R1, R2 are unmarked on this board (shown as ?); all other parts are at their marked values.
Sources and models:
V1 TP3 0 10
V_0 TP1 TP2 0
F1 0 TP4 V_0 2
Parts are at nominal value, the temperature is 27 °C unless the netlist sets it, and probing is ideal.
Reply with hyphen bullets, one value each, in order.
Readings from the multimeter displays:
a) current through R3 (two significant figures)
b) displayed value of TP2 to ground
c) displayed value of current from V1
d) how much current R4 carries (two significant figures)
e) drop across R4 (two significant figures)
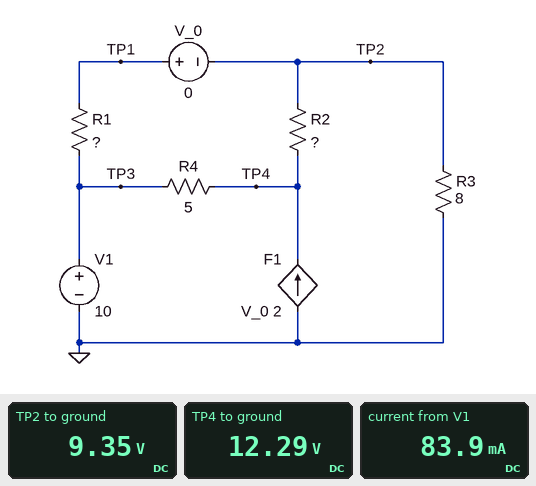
- 1.2 A
- 9.35 V
- 83.9 mA
- 460 mA
- 2.3 V
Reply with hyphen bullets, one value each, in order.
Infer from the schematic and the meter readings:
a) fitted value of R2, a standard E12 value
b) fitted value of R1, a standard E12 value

- 4.7 Ω
- 1.2 Ω
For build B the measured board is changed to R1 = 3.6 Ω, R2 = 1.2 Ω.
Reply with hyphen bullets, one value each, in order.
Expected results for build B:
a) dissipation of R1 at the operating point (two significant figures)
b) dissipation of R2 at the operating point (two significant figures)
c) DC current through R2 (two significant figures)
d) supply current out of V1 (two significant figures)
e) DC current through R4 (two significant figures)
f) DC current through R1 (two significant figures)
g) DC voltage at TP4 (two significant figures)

- 420 mW
- 680 mW
- 750 mA
- 410 mA
- 66 mA
- 340 mA
- 9.7 V
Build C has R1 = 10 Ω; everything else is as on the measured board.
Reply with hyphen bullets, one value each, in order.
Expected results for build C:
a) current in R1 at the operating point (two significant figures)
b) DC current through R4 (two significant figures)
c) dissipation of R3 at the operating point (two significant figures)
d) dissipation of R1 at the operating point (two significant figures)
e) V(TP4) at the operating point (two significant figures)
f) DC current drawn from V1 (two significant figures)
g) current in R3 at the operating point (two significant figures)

- 290 mA
- 18 mA
- 6.3 W
- 840 mW
- 9.9 V
- 310 mA
- 890 mA
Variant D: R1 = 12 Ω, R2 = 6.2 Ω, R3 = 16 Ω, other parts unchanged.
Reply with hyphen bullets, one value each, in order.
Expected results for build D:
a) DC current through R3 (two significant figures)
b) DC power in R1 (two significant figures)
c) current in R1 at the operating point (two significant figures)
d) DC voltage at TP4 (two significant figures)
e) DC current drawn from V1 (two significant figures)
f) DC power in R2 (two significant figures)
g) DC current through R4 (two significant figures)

- 500 mA
- 340 mW
- 170 mA
- 10 V
- 160 mA
- 680 mW
- 6.0 mA
